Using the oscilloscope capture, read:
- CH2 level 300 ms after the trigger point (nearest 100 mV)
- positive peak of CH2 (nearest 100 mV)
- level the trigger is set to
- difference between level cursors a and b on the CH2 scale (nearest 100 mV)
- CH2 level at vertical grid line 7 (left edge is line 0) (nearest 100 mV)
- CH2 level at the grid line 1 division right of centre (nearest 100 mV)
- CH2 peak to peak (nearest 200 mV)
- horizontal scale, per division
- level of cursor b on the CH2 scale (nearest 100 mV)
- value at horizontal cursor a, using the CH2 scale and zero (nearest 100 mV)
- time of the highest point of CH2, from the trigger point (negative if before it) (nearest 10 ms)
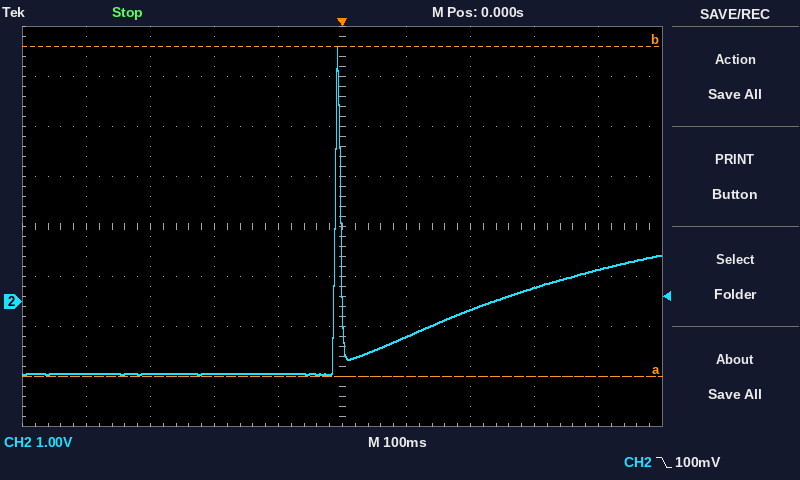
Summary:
300 mV
5.1 V
100 mV
6.6 V
-200 mV
-700 mV
6.6 V
100 ms
5.1 V
-1.5 V
-10 ms
